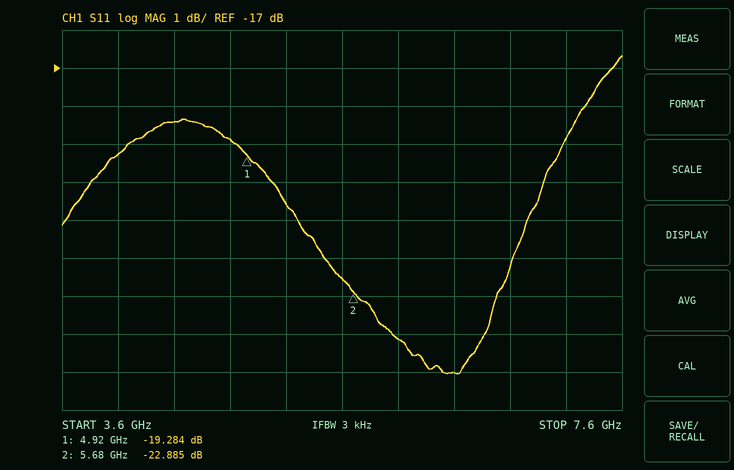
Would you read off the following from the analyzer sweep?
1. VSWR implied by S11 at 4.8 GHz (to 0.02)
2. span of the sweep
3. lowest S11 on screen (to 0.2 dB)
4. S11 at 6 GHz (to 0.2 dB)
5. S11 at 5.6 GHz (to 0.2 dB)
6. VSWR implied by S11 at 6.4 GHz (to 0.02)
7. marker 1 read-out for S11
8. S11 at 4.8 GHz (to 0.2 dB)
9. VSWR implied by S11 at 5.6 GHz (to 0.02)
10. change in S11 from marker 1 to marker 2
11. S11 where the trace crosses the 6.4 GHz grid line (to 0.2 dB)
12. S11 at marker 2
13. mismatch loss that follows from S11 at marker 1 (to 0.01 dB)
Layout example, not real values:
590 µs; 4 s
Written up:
1.26; 4 GHz; -25.0 dB; -24.2 dB; -22.6 dB; 1.12; -19.284 dB; -18.8 dB; 1.16; -3.601 dB; -25.0 dB; -22.885 dB; 0.05 dB
